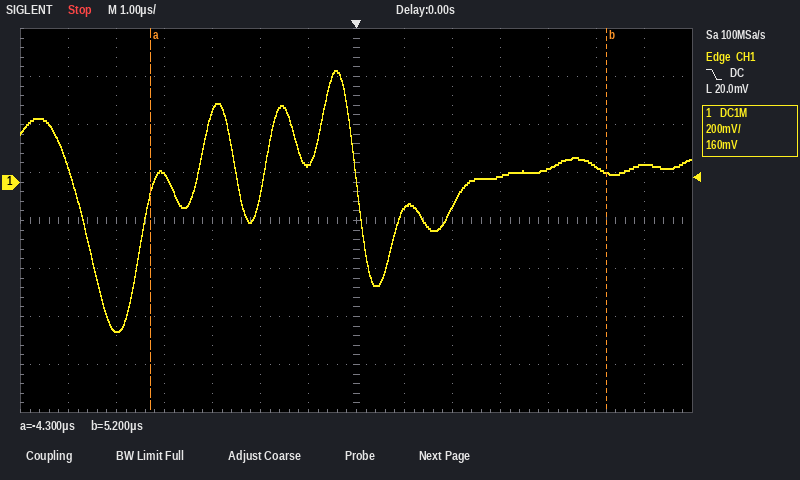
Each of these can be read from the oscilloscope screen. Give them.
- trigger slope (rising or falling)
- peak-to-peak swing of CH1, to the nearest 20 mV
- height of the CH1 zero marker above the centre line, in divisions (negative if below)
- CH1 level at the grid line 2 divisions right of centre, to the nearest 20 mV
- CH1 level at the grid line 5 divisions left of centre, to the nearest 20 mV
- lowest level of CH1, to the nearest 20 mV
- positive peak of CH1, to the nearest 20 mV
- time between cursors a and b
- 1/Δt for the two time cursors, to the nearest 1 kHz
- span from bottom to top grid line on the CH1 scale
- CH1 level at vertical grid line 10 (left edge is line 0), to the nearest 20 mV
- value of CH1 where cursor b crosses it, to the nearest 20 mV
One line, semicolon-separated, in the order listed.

falling; 1.08 V; +0.8 div; -100 mV; -620 mV; -620 mV; 460 mV; 9.5 µs; 105 kHz; 1.6 V; 20 mV; 40 mV
